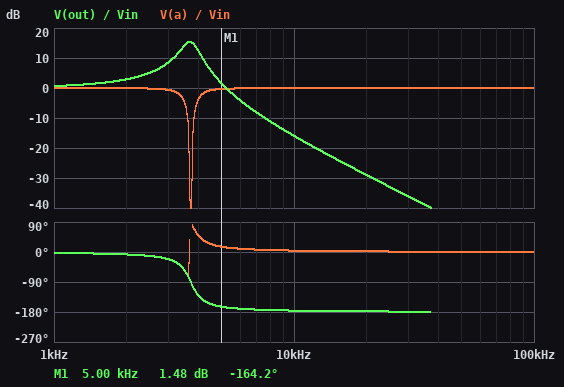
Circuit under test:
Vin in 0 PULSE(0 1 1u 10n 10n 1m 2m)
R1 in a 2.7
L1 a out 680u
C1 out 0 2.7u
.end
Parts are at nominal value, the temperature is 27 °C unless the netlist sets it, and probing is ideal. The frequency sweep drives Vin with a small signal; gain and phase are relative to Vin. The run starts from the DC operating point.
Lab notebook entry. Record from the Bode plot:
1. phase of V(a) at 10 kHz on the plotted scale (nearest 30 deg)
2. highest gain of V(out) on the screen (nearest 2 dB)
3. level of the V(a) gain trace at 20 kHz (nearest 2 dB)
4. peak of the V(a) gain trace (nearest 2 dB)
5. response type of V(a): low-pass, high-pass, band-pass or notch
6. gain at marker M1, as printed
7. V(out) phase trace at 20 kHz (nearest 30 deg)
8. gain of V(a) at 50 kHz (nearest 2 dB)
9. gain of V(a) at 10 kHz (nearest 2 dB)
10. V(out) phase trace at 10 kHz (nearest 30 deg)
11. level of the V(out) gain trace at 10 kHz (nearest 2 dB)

0 deg
16 dB
0 dB
0 dB
notch
1.48 dB
-180 deg
0 dB
0 dB
-180 deg
-16 dB
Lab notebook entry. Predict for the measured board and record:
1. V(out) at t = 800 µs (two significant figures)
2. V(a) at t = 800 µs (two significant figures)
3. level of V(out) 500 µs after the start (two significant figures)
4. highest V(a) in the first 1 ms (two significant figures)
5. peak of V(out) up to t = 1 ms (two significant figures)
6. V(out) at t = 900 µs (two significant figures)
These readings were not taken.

810 mV
1.0 V
810 mV
1.1 V
1.8 V
1.1 V
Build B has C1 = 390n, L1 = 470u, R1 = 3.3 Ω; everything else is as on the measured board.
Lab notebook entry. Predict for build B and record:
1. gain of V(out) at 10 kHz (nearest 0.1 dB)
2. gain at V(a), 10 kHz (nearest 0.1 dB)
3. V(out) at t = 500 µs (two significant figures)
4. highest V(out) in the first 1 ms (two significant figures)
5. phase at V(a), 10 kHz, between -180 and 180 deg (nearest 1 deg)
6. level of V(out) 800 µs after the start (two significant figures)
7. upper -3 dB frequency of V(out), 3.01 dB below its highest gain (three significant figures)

10.8 dB
-0.4 dB
900 mV
1.9 V
-16 deg
1.0 V
12.3 kHz
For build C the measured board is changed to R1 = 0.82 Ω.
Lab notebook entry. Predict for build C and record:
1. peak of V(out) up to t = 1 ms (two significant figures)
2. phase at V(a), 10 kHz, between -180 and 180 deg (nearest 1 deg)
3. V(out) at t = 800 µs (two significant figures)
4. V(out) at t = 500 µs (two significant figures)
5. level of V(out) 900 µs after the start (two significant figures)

1.9 V
1 deg
400 mV
570 mV
1.3 V
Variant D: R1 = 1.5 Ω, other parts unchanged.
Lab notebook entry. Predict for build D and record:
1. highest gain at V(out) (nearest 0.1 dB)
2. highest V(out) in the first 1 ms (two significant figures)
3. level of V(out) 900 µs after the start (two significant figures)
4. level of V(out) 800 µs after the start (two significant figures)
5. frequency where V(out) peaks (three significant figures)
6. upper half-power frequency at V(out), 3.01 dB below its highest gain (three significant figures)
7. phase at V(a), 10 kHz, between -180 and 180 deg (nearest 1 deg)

20.5 dB
1.9 V
1.2 V
600 mV
3.71 kHz
3.88 kHz
2 deg
